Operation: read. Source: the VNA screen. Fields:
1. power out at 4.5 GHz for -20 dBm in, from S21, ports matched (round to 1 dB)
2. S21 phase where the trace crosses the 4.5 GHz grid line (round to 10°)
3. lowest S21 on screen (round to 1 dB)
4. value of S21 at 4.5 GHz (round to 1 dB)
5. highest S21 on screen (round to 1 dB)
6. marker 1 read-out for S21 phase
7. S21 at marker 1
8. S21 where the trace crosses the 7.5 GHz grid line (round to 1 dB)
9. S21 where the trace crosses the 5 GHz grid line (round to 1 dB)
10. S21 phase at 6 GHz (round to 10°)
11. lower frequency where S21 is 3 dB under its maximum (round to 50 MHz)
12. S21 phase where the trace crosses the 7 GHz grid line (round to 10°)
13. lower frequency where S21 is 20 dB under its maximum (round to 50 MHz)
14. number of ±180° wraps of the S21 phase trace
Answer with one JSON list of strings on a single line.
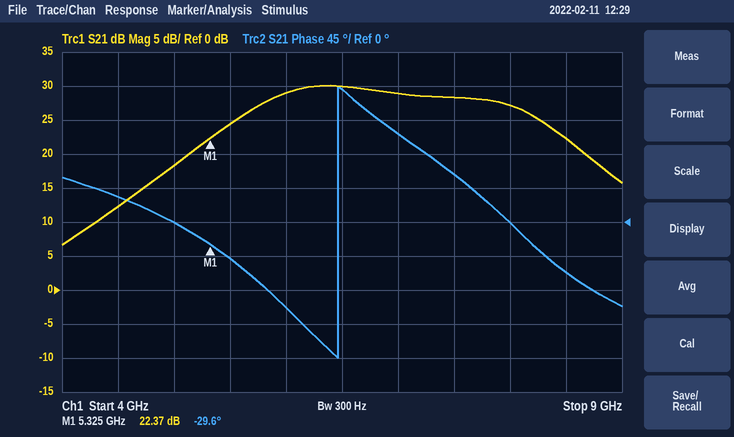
["-8 dBm", "30°", "7 dB", "12 dB", "30 dB", "-29.6°", "22.37 dB", "28 dB", "18 dB", "-110°", "5.75 GHz", "120°", "4.30 GHz", "1"]
